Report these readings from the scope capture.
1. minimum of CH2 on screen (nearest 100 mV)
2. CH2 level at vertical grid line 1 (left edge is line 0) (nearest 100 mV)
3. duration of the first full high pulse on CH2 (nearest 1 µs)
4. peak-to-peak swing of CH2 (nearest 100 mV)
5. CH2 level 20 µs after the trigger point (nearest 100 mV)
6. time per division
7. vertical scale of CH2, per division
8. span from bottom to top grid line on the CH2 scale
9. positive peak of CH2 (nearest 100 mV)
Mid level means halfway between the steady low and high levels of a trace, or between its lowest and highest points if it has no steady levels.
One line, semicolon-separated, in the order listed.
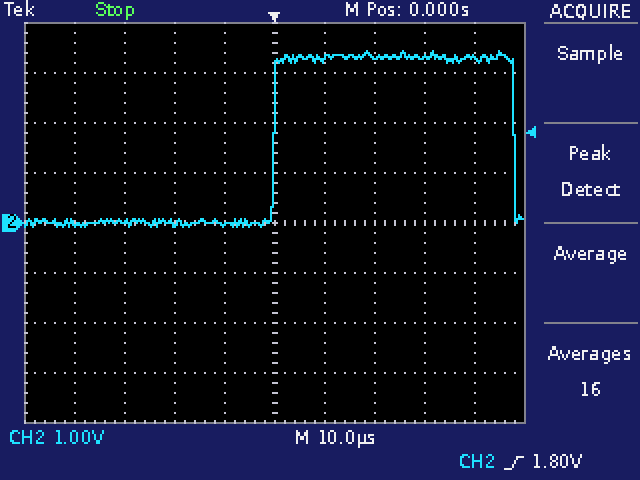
-100 mV; 0.0 V; 48 µs; 3.5 V; 3.3 V; 10 µs; 1 V; 8 V; 3.4 V
